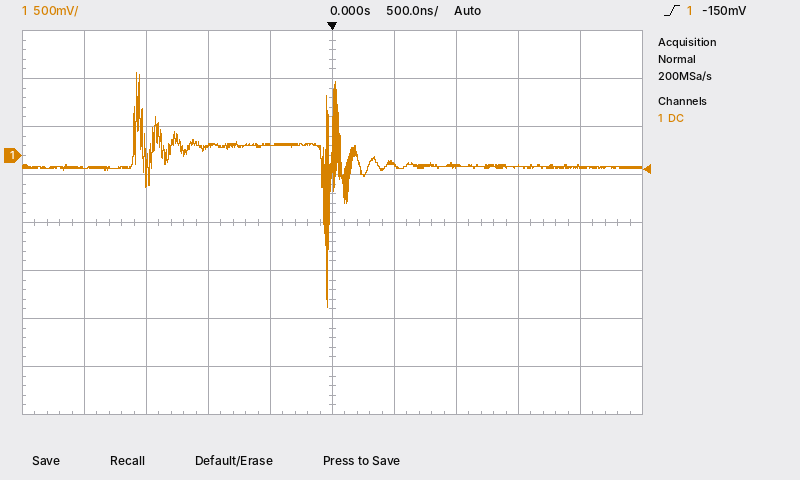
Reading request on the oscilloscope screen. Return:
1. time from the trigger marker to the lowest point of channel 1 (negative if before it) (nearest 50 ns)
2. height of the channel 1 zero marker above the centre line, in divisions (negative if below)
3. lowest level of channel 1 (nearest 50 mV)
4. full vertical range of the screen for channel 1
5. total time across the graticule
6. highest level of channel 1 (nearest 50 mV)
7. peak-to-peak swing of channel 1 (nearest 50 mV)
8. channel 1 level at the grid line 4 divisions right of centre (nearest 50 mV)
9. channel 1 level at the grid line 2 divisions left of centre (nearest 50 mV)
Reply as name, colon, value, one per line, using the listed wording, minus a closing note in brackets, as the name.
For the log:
time from the trigger marker to the lowest point of channel 1 (negative if before it): -50 ns
height of the channel 1 zero marker above the centre line, in divisions: +1.4 div
lowest level of channel 1: -1.60 V
full vertical range of the screen for channel 1: 4 V
total time across the graticule: 5 µs
highest level of channel 1: 850 mV
peak-to-peak swing of channel 1: 2.45 V
channel 1 level at the grid line 4 divisions right of centre: -100 mV
channel 1 level at the grid line 2 divisions left of centre: 100 mV
